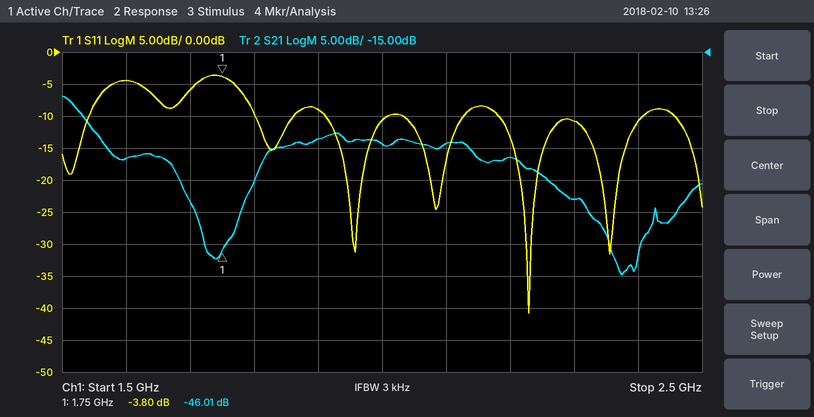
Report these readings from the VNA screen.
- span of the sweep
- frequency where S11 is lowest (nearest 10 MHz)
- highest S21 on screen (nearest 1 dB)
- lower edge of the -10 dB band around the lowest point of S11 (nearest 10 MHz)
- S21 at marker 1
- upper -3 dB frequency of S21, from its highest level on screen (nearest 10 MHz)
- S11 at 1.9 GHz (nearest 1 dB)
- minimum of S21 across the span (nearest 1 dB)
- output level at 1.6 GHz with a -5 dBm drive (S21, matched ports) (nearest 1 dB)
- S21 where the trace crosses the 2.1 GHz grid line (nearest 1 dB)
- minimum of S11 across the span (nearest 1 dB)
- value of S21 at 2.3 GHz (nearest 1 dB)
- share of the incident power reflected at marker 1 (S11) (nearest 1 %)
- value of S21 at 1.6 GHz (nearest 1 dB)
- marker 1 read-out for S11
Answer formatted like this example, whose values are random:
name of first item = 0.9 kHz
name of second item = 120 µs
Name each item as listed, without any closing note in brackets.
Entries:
span of the sweep = 1 GHz
frequency where S11 is lowest = 2.23 GHz
highest S21 on screen = -22 dB
lower edge of the -10 dB band around the lowest point of S11 = 2.18 GHz
S21 at marker 1 = -46.01 dB
upper -3 dB frequency of S21, from its highest level on screen = 1.53 GHz
S11 at 1.9 GHz = -9 dB
minimum of S21 across the span = -50 dB
output level at 1.6 GHz with a -5 dBm drive (S21, matched ports) = -37 dBm
S21 where the trace crosses the 2.1 GHz grid line = -29 dB
minimum of S11 across the span = -41 dB
value of S21 at 2.3 GHz = -38 dB
share of the incident power reflected at marker 1 (S11) = 42 %
value of S21 at 1.6 GHz = -32 dB
marker 1 read-out for S11 = -3.80 dB
